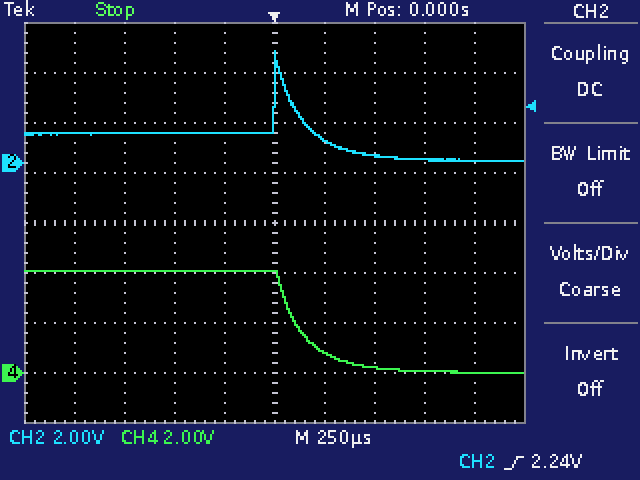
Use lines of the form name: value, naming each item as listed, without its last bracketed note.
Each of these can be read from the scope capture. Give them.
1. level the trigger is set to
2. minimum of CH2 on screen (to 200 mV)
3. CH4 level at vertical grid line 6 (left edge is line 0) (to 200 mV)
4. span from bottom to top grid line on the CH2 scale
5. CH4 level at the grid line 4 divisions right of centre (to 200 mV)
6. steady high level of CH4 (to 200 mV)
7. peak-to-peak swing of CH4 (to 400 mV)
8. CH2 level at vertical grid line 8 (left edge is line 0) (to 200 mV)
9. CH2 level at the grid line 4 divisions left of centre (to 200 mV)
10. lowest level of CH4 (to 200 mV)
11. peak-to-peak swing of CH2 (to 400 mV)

level the trigger is set to: 2.24 V
minimum of CH2 on screen: 0.0 V
CH4 level at vertical grid line 6 (left edge is line 0): 800 mV
span from bottom to top grid line on the CH2 scale: 16 V
CH4 level at the grid line 4 divisions right of centre: 0.0 V
steady high level of CH4: 4.0 V
peak-to-peak swing of CH4: 4.0 V
CH2 level at vertical grid line 8 (left edge is line 0): 200 mV
CH2 level at the grid line 4 divisions left of centre: 1.2 V
lowest level of CH4: 0.0 V
peak-to-peak swing of CH2: 4.4 V
